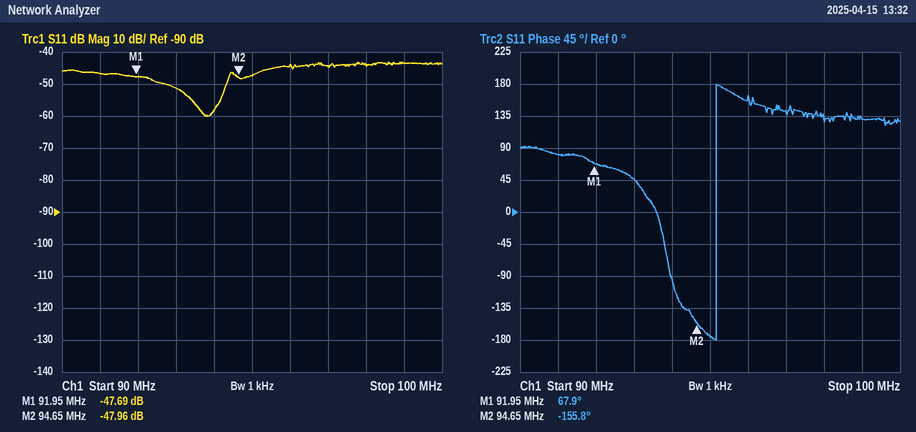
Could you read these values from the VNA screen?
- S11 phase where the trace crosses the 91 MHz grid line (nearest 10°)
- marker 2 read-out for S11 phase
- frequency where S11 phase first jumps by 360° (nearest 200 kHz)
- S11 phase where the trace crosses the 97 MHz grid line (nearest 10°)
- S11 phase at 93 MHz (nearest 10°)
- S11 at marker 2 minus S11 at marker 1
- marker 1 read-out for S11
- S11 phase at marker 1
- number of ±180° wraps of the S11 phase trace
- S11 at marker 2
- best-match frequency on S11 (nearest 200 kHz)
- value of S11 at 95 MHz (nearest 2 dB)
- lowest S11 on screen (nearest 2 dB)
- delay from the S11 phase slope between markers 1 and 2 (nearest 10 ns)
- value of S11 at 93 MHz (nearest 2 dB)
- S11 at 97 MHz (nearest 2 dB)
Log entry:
80°
-155.8°
95.2 MHz
140°
50°
-0.27 dB
-47.69 dB
67.9°
1
-47.96 dB
93.8 MHz
-48 dB
-60 dB
230 ns
-52 dB
-44 dB
